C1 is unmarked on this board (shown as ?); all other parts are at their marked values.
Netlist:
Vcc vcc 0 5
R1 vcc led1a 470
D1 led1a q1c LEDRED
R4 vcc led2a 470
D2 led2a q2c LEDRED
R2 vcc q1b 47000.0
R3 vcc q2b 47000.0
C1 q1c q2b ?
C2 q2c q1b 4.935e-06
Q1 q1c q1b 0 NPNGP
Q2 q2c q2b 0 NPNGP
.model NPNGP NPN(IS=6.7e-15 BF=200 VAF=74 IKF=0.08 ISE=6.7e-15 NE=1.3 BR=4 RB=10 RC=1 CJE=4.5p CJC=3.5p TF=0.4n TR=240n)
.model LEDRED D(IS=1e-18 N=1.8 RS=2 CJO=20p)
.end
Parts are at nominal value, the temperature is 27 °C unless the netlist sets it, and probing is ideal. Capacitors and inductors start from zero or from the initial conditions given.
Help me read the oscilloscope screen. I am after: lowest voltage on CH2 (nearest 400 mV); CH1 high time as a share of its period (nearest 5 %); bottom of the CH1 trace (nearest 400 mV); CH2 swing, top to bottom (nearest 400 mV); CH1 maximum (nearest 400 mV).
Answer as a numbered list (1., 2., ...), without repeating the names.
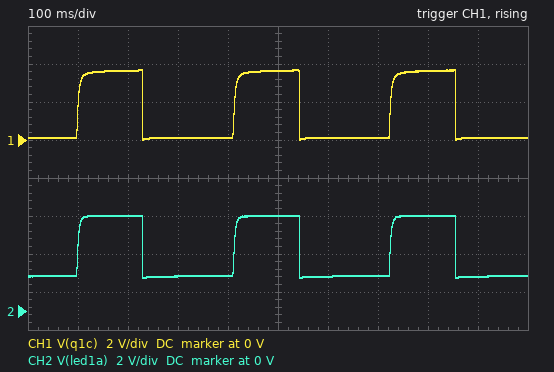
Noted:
1. 1.6 V
2. 40 %
3. 0 V
4. 3.2 V
5. 3.6 V
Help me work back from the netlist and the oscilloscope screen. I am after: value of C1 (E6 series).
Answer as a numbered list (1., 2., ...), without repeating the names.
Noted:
1. 6.8 µF
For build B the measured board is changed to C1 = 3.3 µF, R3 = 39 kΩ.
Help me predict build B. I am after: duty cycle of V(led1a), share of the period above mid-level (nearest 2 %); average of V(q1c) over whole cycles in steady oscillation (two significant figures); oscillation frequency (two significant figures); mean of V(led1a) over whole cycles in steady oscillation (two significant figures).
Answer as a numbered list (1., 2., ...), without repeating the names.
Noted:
1. 64 %
2. 2.3 V
3. 4.9 Hz
4. 3.8 V
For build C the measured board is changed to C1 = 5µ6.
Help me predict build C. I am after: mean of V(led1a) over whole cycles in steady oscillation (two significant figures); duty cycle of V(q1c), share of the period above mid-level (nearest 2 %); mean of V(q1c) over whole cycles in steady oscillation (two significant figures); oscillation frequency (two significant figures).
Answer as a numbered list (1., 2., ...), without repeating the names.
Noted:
1. 3.3 V
2. 46 %
3. 1.7 V
4. 3.6 Hz
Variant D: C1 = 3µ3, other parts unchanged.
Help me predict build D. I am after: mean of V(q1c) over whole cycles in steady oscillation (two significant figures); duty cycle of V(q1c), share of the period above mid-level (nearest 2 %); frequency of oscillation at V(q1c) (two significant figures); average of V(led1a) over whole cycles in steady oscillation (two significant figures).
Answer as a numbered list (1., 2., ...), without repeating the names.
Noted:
1. 2.2 V
2. 60 %
3. 4.6 Hz
4. 3.7 V
